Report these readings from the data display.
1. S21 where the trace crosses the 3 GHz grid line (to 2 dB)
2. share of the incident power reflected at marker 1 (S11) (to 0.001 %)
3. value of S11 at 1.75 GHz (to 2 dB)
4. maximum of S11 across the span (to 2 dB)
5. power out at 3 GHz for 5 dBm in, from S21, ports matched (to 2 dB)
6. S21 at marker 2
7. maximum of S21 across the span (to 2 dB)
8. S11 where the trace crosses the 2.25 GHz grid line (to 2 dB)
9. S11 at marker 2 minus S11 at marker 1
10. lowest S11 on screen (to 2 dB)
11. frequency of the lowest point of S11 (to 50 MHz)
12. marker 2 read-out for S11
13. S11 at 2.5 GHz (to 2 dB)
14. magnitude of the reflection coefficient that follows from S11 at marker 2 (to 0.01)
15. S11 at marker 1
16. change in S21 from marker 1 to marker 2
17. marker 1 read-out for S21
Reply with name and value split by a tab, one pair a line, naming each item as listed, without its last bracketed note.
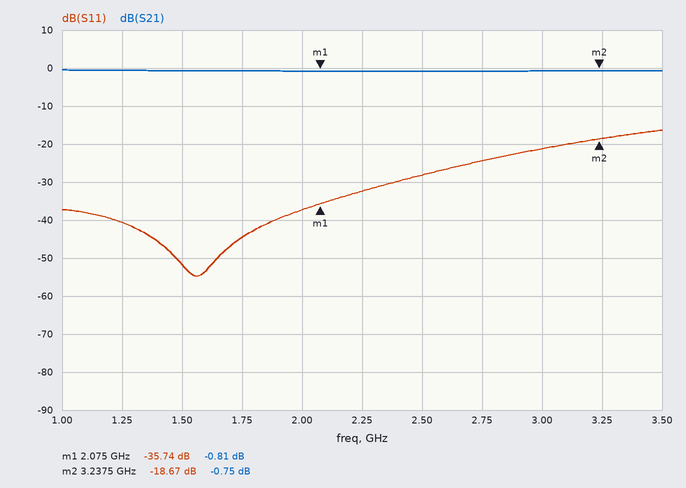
S21 where the trace crosses the 3 GHz grid line	0 dB
share of the incident power reflected at marker 1 (S11)	0.027 %
value of S11 at 1.75 GHz	-44 dB
maximum of S11 across the span	-16 dB
power out at 3 GHz for 5 dBm in, from S21, ports matched	4 dBm
S21 at marker 2	-0.75 dB
maximum of S21 across the span	0 dB
S11 where the trace crosses the 2.25 GHz grid line	-32 dB
S11 at marker 2 minus S11 at marker 1	17.07 dB
lowest S11 on screen	-54 dB
frequency of the lowest point of S11	1.55 GHz
marker 2 read-out for S11	-18.67 dB
S11 at 2.5 GHz	-28 dB
magnitude of the reflection coefficient that follows from S11 at marker 2	0.12
S11 at marker 1	-35.74 dB
change in S21 from marker 1 to marker 2	0.06 dB
marker 1 read-out for S21	-0.81 dB
